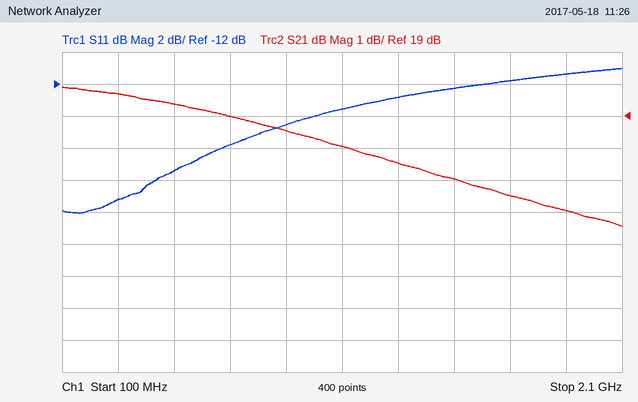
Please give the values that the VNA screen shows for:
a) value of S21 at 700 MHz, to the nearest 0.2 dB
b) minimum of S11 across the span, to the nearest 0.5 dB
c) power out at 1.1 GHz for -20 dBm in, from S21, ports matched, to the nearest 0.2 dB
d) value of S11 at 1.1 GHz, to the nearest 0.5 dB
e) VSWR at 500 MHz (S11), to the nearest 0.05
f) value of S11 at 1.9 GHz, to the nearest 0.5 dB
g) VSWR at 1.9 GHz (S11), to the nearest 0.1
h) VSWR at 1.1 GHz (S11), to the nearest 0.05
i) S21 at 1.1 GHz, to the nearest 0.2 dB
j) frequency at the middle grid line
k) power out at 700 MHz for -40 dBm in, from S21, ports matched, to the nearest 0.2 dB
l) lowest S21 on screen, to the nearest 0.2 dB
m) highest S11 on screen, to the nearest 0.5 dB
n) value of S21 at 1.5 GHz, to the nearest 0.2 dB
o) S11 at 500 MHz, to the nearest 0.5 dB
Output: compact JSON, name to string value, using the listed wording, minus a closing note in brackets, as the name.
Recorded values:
{"value of S21 at 700 MHz, to the nearest 0.2 dB": "19.0 dB", "minimum of S11 across the span, to the nearest 0.5 dB": "-20.0 dB", "power out at 1.1 GHz for -20 dBm in, from S21, ports matched, to the nearest 0.2 dB": "-2.0 dBm", "value of S11 at 1.1 GHz, to the nearest 0.5 dB": "-13.5 dB", "VSWR at 500 MHz (S11), to the nearest 0.05": "1.30", "value of S11 at 1.9 GHz, to the nearest 0.5 dB": "-11.5 dB", "VSWR at 1.9 GHz (S11), to the nearest 0.1": "1.7", "VSWR at 1.1 GHz (S11), to the nearest 0.05": "1.55", "S21 at 1.1 GHz, to the nearest 0.2 dB": "18.0 dB", "frequency at the middle grid line": "1.1 GHz", "power out at 700 MHz for -40 dBm in, from S21, ports matched, to the nearest 0.2 dB": "-21.0 dBm", "lowest S21 on screen, to the nearest 0.2 dB": "15.6 dB", "highest S11 on screen, to the nearest 0.5 dB": "-11.0 dB", "value of S21 at 1.5 GHz, to the nearest 0.2 dB": "17.0 dB", "S11 at 500 MHz, to the nearest 0.5 dB": "-17.5 dB"}
